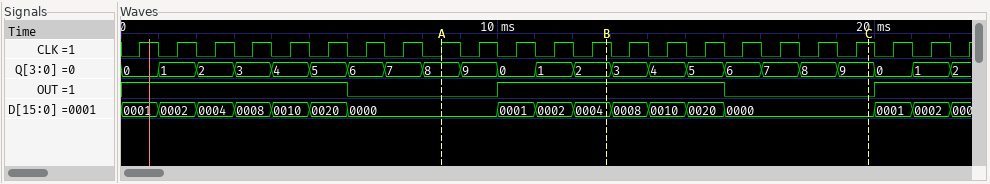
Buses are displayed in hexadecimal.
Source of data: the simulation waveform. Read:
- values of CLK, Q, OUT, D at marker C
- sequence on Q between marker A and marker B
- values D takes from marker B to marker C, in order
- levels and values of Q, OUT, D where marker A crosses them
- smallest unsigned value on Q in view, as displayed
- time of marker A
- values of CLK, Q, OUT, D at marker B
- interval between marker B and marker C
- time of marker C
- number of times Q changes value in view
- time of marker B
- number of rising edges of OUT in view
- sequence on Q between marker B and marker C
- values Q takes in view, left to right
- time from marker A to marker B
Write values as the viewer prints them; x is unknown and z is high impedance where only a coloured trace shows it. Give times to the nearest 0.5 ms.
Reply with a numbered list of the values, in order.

1. CLK=1, Q=9, OUT=0, D=0000
2. 8, 9, 0, 1, 2
3. 0004, 0008, 0010, 0020, 0000
4. Q=8, OUT=0, D=0000
5. 0
6. 8.5 ms
7. CLK=1, Q=2, OUT=1, D=0004
8. 7 ms
9. 20 ms
10. 22
11. 13 ms
12. 2
13. 2, 3, 4, 5, 6, 7, 8, 9
14. 0, 1, 2, 3, 4, 5, 6, 7, 8, 9, 0, 1, 2, 3, 4, 5, 6, 7, 8, 9, 0, 1, 2
15. 4.5 ms
